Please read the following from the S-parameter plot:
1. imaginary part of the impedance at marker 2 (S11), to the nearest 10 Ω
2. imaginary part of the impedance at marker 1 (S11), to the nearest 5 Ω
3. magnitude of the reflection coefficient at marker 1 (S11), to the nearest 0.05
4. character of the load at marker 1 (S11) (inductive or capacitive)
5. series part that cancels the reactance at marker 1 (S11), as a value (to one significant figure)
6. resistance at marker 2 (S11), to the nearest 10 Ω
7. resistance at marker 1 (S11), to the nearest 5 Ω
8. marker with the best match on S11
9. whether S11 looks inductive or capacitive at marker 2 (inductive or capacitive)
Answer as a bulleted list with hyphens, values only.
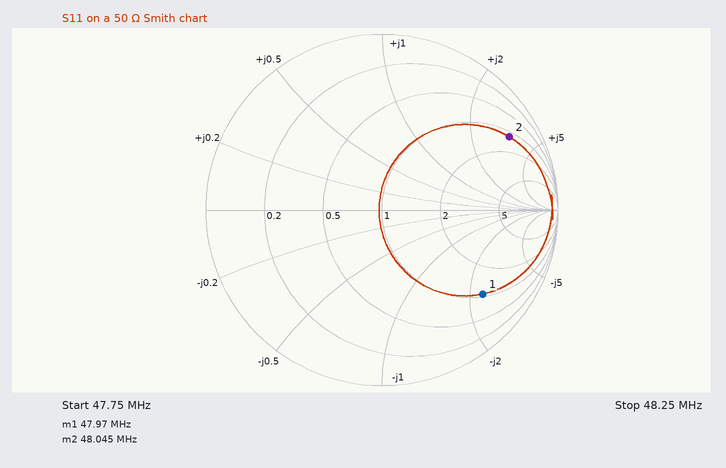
- +170 Ω
- -115 Ω
- 0.75
- capacitive
- 400 nH
- 60 Ω
- 55 Ω
- marker 1
- inductive
